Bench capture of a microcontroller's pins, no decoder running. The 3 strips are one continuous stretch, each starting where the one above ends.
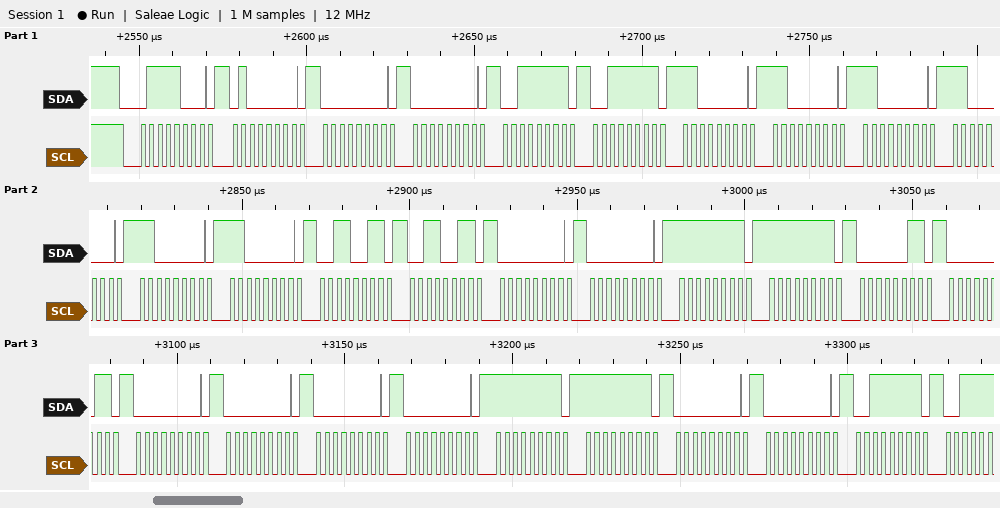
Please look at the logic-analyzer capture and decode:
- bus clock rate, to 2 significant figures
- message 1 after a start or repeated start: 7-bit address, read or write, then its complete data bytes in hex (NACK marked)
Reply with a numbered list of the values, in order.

1. 400 kHz
2. 0x3C write: 40 00 00 3F 3F C0 C0 C0 C0 C0 C0 33 33 00 00 FF FF 03 03 00 00 00 00 FF FF 00 00 3F
